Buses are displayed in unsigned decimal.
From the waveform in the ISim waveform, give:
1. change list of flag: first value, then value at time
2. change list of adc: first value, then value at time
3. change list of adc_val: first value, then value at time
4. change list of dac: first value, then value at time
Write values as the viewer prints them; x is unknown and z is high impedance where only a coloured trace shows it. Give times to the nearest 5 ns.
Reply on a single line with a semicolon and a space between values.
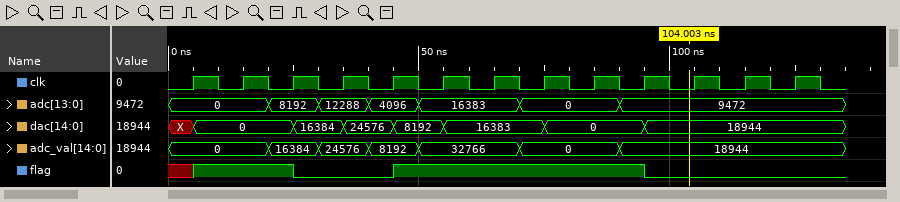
x, 1 at 5 ns, 0 at 25 ns, 1 at 45 ns, 0 at 95 ns; 0, 8192 at 20 ns, 12288 at 30 ns, 4096 at 40 ns, 16383 at 50 ns, 0 at 70 ns, 9472 at 90 ns; 0, 16384 at 20 ns, 24576 at 30 ns, 8192 at 40 ns, 32766 at 50 ns, 0 at 70 ns, 18944 at 90 ns; X, 0 at 5 ns, 16384 at 25 ns, 24576 at 35 ns, 8192 at 45 ns, 16383 at 55 ns, 0 at 75 ns, 18944 at 95 ns
